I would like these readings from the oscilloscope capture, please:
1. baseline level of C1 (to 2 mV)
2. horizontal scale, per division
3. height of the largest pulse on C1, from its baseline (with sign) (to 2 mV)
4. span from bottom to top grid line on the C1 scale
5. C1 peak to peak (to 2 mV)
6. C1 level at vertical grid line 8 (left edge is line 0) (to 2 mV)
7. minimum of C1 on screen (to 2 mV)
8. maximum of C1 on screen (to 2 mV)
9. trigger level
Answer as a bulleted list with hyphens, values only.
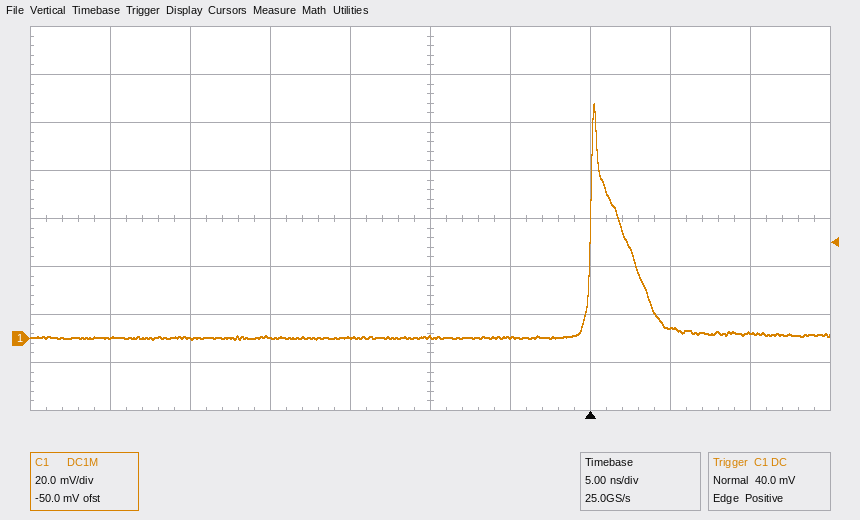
- 0 mV
- 5 ns
- +98 mV
- 160 mV
- 98 mV
- 4 mV
- 0 mV
- 98 mV
- 40.0 mV
